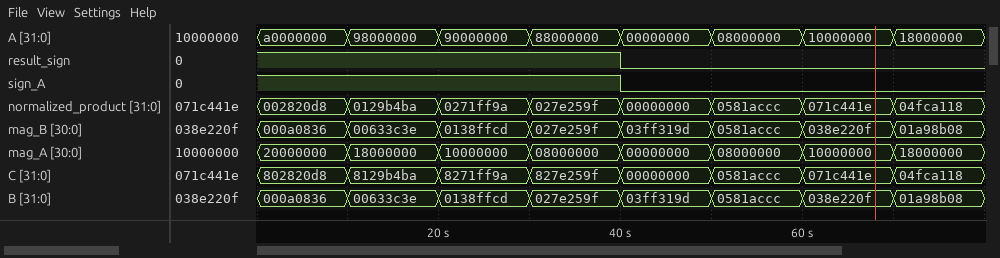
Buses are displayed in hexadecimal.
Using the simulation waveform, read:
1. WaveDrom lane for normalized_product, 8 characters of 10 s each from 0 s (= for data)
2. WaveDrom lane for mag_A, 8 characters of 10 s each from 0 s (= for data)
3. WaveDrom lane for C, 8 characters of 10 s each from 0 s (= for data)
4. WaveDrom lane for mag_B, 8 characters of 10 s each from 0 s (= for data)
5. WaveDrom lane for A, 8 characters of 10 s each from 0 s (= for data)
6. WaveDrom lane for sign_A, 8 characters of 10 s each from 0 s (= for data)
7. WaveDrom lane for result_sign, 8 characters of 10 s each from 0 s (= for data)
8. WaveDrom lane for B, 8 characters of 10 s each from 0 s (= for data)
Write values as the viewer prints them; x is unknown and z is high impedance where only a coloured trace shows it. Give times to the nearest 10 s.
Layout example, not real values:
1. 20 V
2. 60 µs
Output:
1. {name: 'normalized_product', wave: '========', data: '002820d8 0129b4ba 0271ff9a 027e259f 00000000 0581accc 071c441e 04fca118'}
2. {name: 'mag_A', wave: '========', data: '20000000 18000000 10000000 08000000 00000000 08000000 10000000 18000000'}
3. {name: 'C', wave: '========', data: '802820d8 8129b4ba 8271ff9a 827e259f 00000000 0581accc 071c441e 04fca118'}
4. {name: 'mag_B', wave: '========', data: '000a0836 00633c3e 0138ffcd 027e259f 03ff319d 0581accc 038e220f 01a98b08'}
5. {name: 'A', wave: '========', data: 'a0000000 98000000 90000000 88000000 00000000 08000000 10000000 18000000'}
6. {name: 'sign_A', wave: '1...0...'}
7. {name: 'result_sign', wave: '1...0...'}
8. {name: 'B', wave: '========', data: '000a0836 00633c3e 0138ffcd 027e259f 03ff319d 0581accc 038e220f 01a98b08'}
